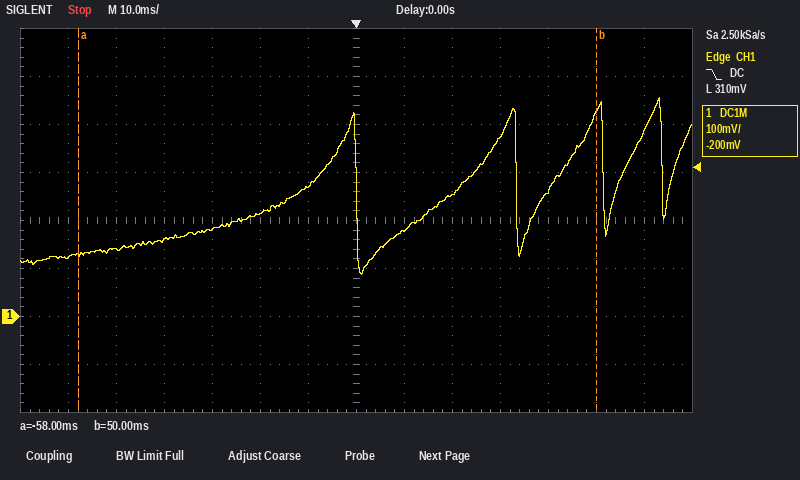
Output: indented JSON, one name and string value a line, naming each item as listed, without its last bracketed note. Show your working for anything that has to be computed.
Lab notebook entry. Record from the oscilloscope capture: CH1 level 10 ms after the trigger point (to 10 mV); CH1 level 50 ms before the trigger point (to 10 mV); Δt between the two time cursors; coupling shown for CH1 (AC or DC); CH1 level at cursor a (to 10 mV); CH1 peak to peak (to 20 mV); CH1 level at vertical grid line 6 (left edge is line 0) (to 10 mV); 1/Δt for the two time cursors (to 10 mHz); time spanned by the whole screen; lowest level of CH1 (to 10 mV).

{
  "CH1 level 10 ms after the trigger point": "180 mV",
  "CH1 level 50 ms before the trigger point": "140 mV",
  "Δt between the two time cursors": "50 ms − (-58 ms) = 108 ms",
  "coupling shown for CH1": "DC",
  "CH1 level at cursor a": "130 mV",
  "CH1 peak to peak": "360 mV",
  "CH1 level at vertical grid line 6 (left edge is line 0)": "270 mV",
  "1/Δt for the two time cursors": "1 / 108 ms ≈ 9.26 Hz",
  "time spanned by the whole screen": "140 ms",
  "lowest level of CH1": "90 mV"
}
